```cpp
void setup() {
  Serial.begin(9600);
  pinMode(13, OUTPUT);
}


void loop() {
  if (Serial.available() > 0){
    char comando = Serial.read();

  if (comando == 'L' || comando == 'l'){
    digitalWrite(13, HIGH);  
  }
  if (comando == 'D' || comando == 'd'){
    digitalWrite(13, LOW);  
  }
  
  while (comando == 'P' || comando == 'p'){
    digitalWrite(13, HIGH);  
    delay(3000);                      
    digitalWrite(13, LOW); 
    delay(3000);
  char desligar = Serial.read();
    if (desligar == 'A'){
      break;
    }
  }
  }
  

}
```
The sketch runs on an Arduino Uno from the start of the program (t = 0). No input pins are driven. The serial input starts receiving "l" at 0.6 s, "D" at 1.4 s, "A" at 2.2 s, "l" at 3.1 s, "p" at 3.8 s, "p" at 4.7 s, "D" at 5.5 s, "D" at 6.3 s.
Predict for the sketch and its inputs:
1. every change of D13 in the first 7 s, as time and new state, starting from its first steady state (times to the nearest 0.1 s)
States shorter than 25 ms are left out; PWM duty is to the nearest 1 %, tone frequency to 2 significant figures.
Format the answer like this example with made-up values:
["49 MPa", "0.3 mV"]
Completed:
["0 s low; 0.6 s high; 1.4 s low; 3.1 s high; 6.8 s low"]
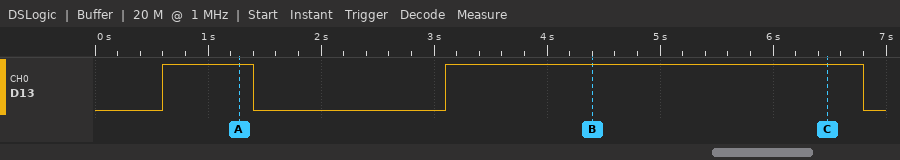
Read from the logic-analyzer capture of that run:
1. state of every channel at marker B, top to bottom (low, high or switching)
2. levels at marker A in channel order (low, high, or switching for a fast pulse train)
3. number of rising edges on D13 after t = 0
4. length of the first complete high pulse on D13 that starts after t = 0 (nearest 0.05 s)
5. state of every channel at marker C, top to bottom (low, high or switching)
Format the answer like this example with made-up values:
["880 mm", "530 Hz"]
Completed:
["D13 high", "D13 high", "2", "0.80 s", "D13 high"]
